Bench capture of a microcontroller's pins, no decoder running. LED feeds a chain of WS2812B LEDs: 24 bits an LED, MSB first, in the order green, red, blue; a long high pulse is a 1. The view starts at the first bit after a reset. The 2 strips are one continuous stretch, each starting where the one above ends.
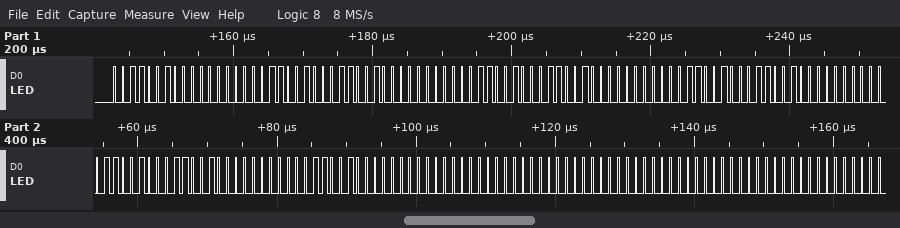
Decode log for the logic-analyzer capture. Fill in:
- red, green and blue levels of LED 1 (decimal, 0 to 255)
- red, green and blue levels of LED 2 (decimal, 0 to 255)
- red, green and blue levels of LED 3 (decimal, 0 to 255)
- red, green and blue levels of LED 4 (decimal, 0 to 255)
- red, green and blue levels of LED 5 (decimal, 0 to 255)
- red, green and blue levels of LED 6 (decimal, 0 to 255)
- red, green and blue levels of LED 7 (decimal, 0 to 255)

0, 50, 50
0, 50, 50
0, 50, 50
0, 50, 50
0, 50, 50
0, 0, 0
0, 0, 0
